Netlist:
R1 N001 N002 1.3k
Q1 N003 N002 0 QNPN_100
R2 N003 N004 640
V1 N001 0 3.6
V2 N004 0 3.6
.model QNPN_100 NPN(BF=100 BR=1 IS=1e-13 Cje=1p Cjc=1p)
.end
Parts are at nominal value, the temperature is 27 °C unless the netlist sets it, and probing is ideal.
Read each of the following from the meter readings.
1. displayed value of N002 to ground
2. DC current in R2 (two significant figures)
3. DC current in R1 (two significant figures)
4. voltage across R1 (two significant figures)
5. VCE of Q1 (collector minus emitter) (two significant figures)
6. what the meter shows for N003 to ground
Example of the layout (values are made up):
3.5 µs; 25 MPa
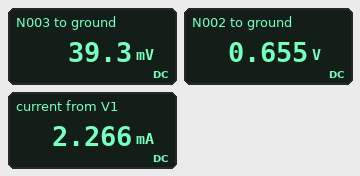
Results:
0.655 V; 5.6 mA; 2.3 mA; 2.9 V; 39 mV; 39.3 mV
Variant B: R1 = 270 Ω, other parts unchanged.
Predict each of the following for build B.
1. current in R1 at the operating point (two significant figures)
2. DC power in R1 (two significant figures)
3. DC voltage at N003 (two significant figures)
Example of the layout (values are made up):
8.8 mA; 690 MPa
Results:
11 mA; 32 mW; 24 mV
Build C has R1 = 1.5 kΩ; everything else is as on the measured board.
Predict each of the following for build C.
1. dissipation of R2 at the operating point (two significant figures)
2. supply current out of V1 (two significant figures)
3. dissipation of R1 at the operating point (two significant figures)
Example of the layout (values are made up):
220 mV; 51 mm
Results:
20 mW; 2.0 mA; 5.8 mW
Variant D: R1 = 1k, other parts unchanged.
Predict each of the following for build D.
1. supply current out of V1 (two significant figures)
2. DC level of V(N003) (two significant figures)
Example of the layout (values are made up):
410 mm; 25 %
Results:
2.9 mA; 36 mV
